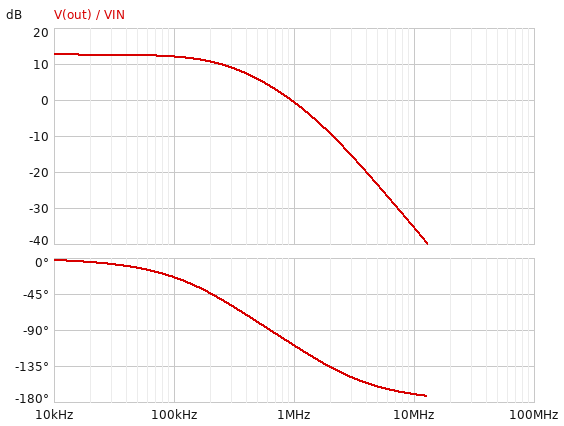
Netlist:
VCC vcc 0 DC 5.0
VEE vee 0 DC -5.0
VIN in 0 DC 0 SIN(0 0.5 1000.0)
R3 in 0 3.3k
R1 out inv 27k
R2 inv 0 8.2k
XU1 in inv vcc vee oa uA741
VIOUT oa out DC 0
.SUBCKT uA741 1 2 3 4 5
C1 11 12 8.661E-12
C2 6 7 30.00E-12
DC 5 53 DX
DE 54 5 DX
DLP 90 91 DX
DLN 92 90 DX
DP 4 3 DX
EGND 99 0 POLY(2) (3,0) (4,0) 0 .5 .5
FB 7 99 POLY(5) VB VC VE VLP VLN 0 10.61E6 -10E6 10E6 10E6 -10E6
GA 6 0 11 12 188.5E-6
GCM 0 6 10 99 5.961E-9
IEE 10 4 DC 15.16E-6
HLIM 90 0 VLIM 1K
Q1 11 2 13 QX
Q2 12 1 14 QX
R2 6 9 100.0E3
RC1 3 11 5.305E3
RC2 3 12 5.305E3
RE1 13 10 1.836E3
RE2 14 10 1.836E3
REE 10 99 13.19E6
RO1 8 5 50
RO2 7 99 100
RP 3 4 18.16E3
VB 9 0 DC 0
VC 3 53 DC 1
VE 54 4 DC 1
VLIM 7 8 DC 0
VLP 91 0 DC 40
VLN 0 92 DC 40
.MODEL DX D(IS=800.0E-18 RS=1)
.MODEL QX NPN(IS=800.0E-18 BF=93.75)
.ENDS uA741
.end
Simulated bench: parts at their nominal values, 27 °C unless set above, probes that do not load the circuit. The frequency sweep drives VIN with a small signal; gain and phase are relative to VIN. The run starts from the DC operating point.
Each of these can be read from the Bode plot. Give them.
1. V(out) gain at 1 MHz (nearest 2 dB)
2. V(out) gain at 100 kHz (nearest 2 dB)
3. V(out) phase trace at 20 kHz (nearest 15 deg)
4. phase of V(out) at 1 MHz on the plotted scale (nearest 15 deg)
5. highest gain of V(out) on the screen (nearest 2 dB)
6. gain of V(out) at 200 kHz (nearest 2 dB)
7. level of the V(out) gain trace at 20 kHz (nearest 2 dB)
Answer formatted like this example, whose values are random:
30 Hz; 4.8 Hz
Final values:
0 dB; 12 dB; 0 deg; -105 deg; 12 dB; 10 dB; 12 dB
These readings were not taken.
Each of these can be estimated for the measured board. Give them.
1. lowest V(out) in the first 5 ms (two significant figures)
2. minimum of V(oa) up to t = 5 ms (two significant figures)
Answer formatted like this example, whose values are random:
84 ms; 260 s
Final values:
-2.1 V; -2.1 V
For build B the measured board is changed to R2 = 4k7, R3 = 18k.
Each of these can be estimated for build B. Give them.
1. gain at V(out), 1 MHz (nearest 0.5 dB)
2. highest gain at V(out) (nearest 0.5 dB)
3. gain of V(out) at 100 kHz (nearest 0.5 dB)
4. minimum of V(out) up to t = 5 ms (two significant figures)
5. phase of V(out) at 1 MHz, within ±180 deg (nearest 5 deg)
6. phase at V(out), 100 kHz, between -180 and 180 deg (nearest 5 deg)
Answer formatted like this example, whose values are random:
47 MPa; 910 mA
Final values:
-1.0 dB; 16.5 dB; 15.0 dB; -3.4 V; -115 deg; -35 deg
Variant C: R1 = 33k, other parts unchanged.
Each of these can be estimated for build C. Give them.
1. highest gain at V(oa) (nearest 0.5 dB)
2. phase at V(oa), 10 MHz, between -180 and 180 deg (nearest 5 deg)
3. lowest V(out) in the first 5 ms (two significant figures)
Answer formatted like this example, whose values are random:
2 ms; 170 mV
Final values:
14.0 dB; -170 deg; -2.5 V
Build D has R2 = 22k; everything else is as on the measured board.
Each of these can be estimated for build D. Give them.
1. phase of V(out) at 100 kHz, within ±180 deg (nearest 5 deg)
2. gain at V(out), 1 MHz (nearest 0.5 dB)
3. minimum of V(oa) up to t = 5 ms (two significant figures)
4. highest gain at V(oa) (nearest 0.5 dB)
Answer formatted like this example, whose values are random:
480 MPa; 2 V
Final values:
-15 deg; 0 dB; -1.1 V; 7.0 dB
